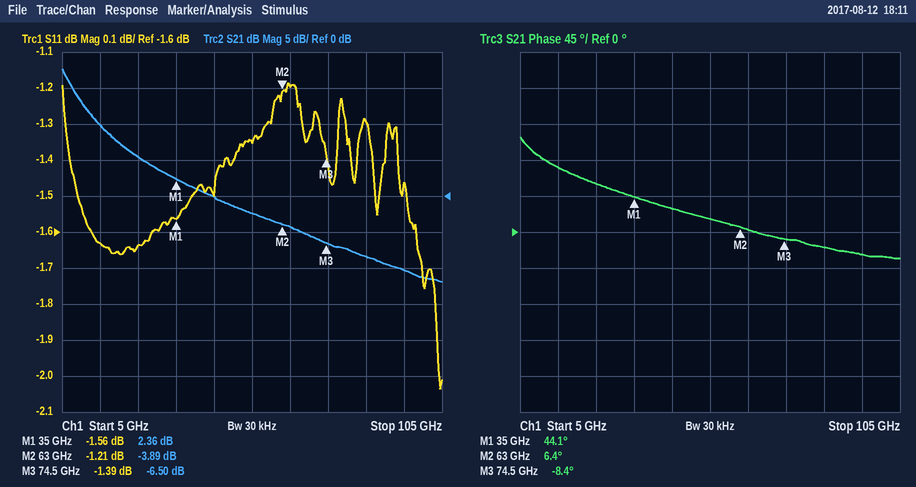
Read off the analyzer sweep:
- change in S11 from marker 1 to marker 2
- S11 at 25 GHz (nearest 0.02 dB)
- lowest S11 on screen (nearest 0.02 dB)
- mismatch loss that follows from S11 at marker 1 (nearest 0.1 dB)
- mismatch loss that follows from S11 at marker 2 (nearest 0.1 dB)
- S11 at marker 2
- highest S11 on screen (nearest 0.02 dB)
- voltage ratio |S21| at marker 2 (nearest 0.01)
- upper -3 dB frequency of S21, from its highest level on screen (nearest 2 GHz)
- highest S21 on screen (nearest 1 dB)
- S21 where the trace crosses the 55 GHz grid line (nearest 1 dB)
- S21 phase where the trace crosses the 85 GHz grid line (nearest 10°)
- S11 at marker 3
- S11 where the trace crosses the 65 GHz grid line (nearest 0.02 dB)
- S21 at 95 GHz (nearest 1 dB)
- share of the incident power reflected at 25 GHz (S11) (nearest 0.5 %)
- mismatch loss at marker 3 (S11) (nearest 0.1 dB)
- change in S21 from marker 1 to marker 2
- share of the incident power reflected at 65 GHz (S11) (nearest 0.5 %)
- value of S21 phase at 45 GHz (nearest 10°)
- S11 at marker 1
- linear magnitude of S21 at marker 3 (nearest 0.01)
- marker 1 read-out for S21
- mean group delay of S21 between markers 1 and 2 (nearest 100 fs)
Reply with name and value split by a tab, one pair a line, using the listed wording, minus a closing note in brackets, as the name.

change in S11 from marker 1 to marker 2	0.35 dB
S11 at 25 GHz	-1.64 dB
lowest S11 on screen	-2.04 dB
mismatch loss that follows from S11 at marker 1	5.2 dB
mismatch loss that follows from S11 at marker 2	6.1 dB
S11 at marker 2	-1.21 dB
highest S11 on screen	-1.18 dB
voltage ratio |S21| at marker 2	0.64
upper -3 dB frequency of S21, from its highest level on screen	8 GHz
highest S21 on screen	18 dB
S21 where the trace crosses the 55 GHz grid line	-2 dB
S21 phase where the trace crosses the 85 GHz grid line	-20°
S11 at marker 3	-1.39 dB
S11 where the trace crosses the 65 GHz grid line	-1.20 dB
S21 at 95 GHz	-10 dB
share of the incident power reflected at 25 GHz (S11)	68.5 %
mismatch loss at marker 3 (S11)	5.6 dB
change in S21 from marker 1 to marker 2	-6.25 dB
share of the incident power reflected at 65 GHz (S11)	76.0 %
value of S21 phase at 45 GHz	30°
S11 at marker 1	-1.56 dB
linear magnitude of S21 at marker 3	0.47
marker 1 read-out for S21	2.36 dB
mean group delay of S21 between markers 1 and 2	3.7 ps
